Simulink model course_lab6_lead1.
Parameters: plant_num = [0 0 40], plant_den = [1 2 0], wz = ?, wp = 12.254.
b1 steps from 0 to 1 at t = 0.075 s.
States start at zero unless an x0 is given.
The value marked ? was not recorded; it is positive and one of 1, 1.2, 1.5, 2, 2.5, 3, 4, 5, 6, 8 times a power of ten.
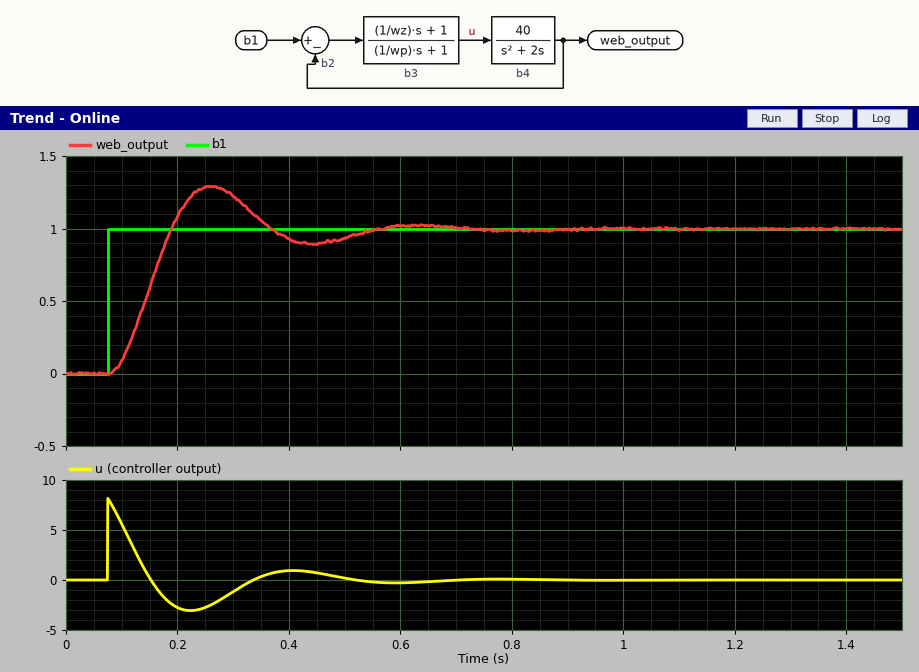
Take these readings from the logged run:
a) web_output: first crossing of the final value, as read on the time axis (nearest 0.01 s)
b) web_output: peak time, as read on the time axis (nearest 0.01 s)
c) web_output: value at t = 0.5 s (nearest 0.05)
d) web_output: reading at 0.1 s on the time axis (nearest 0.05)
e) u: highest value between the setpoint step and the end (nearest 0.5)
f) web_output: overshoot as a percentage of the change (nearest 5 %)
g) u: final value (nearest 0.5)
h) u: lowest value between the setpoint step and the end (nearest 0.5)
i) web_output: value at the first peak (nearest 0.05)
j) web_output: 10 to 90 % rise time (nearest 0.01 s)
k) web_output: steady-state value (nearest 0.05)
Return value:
0.19 s
0.26 s
0.95
0.10
8.0
30 %
0.0
-3.0
1.30
0.08 s
1.00
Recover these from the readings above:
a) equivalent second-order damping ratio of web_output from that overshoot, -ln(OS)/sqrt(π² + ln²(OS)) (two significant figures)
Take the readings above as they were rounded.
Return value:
0.36
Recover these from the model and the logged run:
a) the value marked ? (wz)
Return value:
1.5
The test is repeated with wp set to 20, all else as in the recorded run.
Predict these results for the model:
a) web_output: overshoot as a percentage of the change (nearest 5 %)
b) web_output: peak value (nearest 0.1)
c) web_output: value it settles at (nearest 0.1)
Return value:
20 %
1.2
1.0
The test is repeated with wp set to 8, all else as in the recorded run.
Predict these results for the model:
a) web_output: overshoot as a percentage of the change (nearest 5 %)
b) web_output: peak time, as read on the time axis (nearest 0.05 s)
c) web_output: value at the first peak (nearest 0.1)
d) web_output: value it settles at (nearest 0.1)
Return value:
35 %
0.30 s
1.4
1.0
